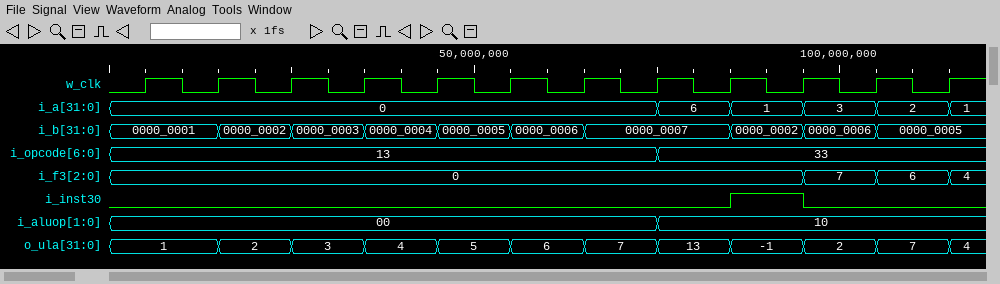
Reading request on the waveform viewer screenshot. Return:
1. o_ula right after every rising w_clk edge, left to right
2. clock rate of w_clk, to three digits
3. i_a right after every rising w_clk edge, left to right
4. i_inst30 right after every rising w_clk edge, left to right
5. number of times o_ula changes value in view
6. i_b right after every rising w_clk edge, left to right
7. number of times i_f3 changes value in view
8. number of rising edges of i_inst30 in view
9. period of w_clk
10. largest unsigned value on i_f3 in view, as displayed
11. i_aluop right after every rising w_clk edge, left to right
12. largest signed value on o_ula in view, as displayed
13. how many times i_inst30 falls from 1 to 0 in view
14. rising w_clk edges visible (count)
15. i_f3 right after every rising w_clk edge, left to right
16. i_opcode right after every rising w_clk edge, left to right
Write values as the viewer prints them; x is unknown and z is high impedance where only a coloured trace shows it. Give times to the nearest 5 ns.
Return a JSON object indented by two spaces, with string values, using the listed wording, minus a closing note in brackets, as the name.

{
  "o_ula right after every rising w_clk edge, left to right": "1, 2, 3, 4, 5, 6, 7, 13, -1, 2, 7, 4",
  "clock rate of w_clk, to three digits": "100 MHz",
  "i_a right after every rising w_clk edge, left to right": "0, 0, 0, 0, 0, 0, 0, 6, 1, 3, 2, 1",
  "i_inst30 right after every rising w_clk edge, left to right": "0 0 0 0 0 0 0 0 1 0 0 0",
  "number of times o_ula changes value in view": "11",
  "i_b right after every rising w_clk edge, left to right": "0000_0001, 0000_0002, 0000_0003, 0000_0004, 0000_0005, 0000_0006, 0000_0007, 0000_0007, 0000_0002, 0000_0006, 0000_0005, 0000_0005",
  "number of times i_f3 changes value in view": "3",
  "number of rising edges of i_inst30 in view": "1",
  "period of w_clk": "10 ns",
  "largest unsigned value on i_f3 in view, as displayed": "7",
  "i_aluop right after every rising w_clk edge, left to right": "00, 00, 00, 00, 00, 00, 00, 10, 10, 10, 10, 10",
  "largest signed value on o_ula in view, as displayed": "13",
  "how many times i_inst30 falls from 1 to 0 in view": "1",
  "rising w_clk edges visible": "12",
  "i_f3 right after every rising w_clk edge, left to right": "0, 0, 0, 0, 0, 0, 0, 0, 0, 7, 6, 4",
  "i_opcode right after every rising w_clk edge, left to right": "13, 13, 13, 13, 13, 13, 13, 33, 33, 33, 33, 33"
}
